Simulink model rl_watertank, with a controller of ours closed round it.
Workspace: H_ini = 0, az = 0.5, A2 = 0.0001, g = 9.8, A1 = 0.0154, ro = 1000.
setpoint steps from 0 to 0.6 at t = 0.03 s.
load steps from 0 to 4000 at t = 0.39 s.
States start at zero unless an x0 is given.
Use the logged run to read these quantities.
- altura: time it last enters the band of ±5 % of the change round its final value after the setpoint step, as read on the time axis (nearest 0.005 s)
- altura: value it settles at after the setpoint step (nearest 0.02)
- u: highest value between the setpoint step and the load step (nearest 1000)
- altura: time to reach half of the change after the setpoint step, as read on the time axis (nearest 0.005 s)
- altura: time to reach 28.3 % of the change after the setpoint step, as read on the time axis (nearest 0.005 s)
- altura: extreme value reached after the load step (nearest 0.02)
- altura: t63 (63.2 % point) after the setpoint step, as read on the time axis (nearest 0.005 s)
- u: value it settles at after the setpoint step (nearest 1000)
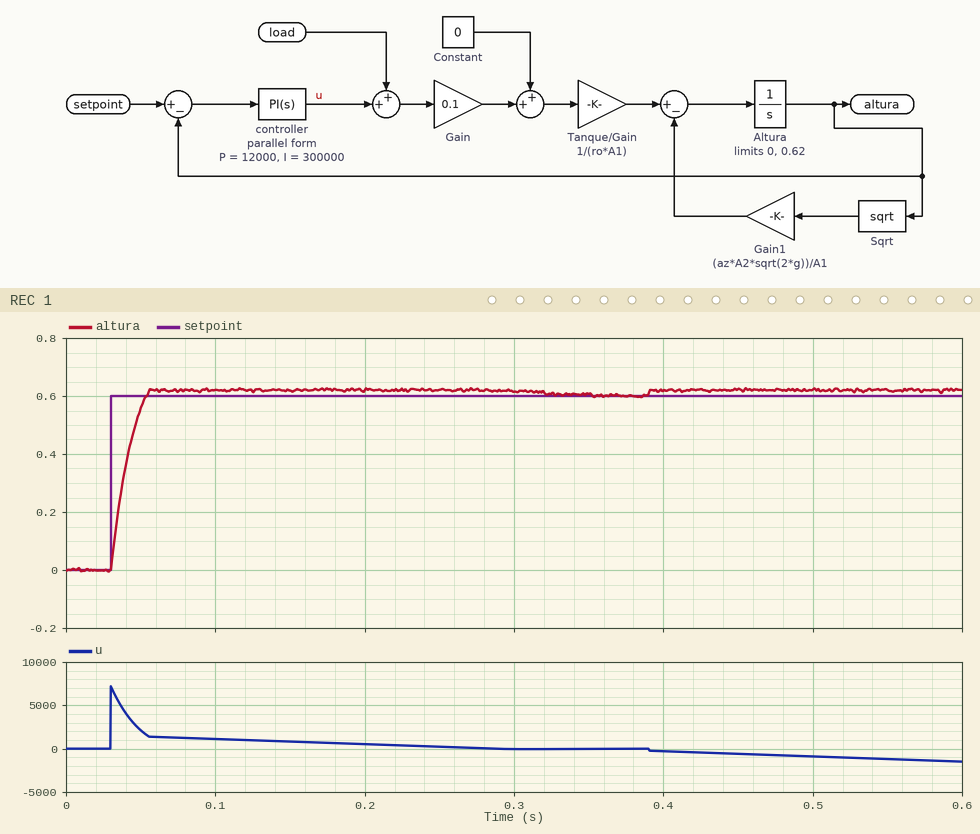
0.050 s
0.60
7000
0.040 s
0.035 s
0.62
0.040 s
0
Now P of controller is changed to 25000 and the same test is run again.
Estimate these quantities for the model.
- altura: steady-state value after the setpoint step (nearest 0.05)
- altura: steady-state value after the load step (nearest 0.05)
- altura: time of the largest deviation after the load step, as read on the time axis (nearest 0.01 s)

0.60
0.60
0.39 s
